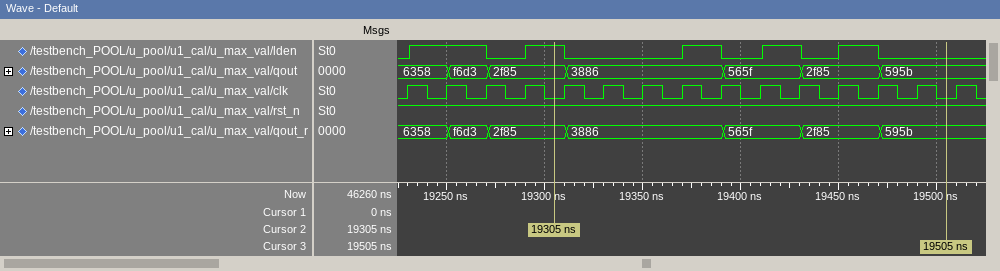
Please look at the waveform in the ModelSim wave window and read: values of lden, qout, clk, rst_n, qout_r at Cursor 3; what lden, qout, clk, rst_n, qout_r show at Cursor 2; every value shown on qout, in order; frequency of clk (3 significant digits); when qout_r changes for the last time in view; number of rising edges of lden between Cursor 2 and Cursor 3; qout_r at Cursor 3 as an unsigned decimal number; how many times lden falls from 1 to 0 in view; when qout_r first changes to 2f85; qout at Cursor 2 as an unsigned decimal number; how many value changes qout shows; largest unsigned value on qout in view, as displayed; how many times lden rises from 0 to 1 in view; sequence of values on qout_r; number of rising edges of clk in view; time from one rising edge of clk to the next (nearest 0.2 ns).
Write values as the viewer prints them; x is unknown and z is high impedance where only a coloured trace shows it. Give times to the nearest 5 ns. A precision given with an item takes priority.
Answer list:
lden=0, qout=595b, clk=0, rst_n=1, qout_r=595b
lden=1, qout=2f85, clk=0, rst_n=1, qout_r=2f85
6358, f6d3, 2f85, 3886, 565f, 2f85, 595b
50.0 MHz
19470 ns
3
22875
5
19270 ns
12165
6
f6d3
5
6358, f6d3, 2f85, 3886, 565f, 2f85, 595b
15
20 ns
